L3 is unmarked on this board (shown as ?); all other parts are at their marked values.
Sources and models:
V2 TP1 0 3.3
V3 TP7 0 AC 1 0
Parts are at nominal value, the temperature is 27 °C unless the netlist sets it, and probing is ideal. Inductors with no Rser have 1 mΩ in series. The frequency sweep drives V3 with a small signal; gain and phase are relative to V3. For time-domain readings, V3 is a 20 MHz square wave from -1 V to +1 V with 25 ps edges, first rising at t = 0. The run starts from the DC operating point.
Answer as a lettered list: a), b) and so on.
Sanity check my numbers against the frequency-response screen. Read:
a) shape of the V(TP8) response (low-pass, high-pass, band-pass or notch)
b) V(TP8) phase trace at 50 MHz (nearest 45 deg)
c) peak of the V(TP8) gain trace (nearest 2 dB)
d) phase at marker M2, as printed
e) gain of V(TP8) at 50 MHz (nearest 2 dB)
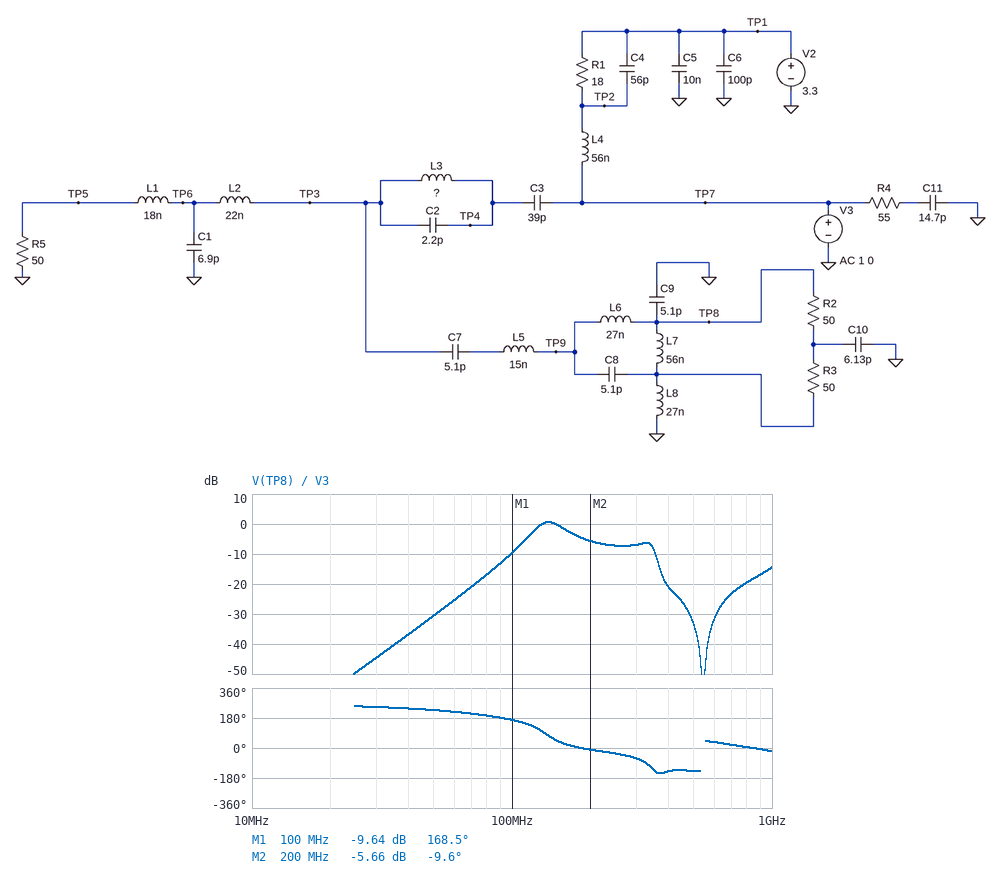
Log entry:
a) band-pass
b) 225 deg
c) 0 dB
d) -9.6 deg
e) -30 dB
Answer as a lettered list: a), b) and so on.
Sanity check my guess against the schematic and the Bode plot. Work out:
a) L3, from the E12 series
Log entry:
a) 39 nH
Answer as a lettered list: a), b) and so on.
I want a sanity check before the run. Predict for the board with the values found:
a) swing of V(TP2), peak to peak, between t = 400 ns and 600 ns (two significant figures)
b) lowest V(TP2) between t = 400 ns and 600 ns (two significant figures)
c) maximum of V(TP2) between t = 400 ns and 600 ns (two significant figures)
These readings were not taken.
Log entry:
a) 2.0 V
b) -1.0 V
c) 1.0 V
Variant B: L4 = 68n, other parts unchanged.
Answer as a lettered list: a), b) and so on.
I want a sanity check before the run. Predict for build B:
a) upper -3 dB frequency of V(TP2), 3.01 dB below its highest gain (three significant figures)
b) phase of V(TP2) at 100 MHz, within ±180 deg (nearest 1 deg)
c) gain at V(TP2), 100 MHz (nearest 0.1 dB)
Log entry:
a) 55.0 MHz
b) -102 deg
c) -7.7 dB
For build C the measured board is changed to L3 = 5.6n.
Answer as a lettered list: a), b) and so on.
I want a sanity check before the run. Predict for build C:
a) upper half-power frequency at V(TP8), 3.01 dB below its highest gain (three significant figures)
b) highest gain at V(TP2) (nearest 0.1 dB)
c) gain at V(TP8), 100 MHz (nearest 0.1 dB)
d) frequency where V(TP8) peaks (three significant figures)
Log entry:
a) 362 MHz
b) 0 dB
c) -11.0 dB
d) 344 MHz
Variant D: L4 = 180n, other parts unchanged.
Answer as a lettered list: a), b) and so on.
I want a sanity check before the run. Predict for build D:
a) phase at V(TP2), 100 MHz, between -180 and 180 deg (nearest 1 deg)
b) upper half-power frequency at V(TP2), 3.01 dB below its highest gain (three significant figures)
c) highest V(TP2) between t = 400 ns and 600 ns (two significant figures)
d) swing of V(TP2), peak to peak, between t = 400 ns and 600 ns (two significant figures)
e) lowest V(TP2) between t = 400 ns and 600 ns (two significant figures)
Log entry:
a) -115 deg
b) 17.7 MHz
c) 870 mV
d) 1.7 V
e) -870 mV
